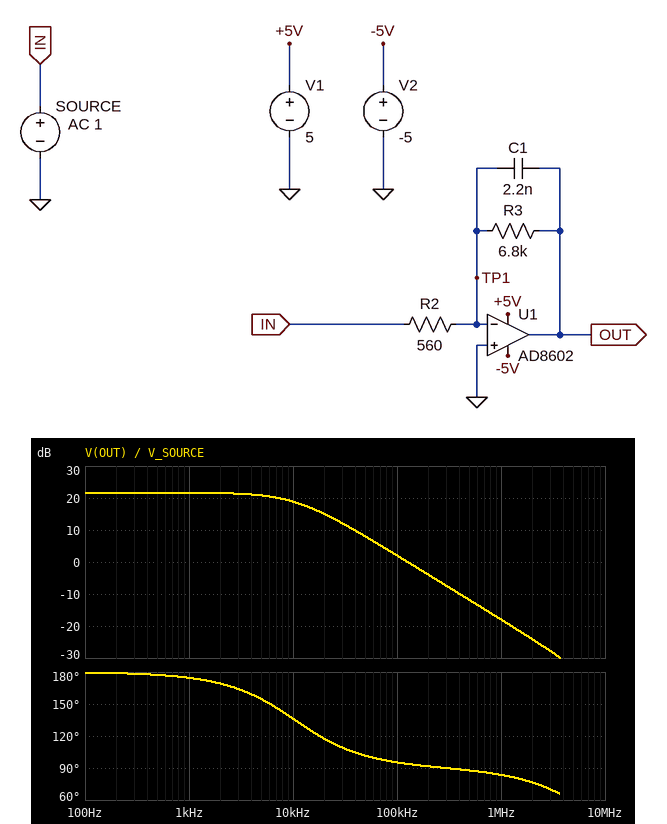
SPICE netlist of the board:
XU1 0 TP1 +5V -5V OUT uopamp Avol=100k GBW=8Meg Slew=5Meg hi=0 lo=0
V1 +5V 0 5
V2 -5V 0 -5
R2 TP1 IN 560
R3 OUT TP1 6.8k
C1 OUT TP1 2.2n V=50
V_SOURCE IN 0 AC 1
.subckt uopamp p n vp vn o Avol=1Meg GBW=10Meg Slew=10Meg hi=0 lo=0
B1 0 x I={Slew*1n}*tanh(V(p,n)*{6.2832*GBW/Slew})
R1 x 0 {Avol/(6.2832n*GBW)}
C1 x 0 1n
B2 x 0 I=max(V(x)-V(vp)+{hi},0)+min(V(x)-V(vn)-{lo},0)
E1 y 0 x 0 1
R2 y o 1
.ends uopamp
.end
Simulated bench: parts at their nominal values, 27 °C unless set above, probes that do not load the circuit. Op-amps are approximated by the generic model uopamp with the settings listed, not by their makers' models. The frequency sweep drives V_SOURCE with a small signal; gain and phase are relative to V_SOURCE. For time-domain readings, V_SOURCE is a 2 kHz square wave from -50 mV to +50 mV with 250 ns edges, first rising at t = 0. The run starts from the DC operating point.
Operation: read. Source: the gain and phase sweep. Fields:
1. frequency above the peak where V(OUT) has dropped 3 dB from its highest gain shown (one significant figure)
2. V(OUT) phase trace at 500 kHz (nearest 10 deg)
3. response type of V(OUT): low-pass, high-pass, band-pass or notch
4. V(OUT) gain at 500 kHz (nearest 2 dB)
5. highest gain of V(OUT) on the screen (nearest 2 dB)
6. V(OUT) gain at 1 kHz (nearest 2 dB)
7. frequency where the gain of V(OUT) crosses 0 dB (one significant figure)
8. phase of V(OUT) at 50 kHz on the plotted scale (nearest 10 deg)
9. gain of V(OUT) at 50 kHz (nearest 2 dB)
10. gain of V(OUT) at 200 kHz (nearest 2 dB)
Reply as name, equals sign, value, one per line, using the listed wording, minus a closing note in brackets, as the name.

frequency above the peak where V(OUT) has dropped 3 dB from its highest gain shown = 10 kHz
V(OUT) phase trace at 500 kHz = 90 deg
response type of V(OUT): low-pass, high-pass, band-pass or notch = low-pass
V(OUT) gain at 500 kHz = -12 dB
highest gain of V(OUT) on the screen = 22 dB
V(OUT) gain at 1 kHz = 22 dB
frequency where the gain of V(OUT) crosses 0 dB = 100 kHz
phase of V(OUT) at 50 kHz on the plotted scale = 100 deg
gain of V(OUT) at 50 kHz = 8 dB
gain of V(OUT) at 200 kHz = -4 dB
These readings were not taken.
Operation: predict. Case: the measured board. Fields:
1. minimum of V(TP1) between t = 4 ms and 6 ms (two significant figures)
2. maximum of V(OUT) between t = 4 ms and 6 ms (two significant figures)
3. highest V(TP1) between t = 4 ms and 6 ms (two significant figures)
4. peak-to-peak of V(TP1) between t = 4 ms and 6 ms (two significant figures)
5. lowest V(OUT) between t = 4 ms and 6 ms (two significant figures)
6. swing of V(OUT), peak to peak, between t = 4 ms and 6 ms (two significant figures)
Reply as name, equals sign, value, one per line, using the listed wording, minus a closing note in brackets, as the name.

minimum of V(TP1) between t = 4 ms and 6 ms = -1.6 mV
maximum of V(OUT) between t = 4 ms and 6 ms = 610 mV
highest V(TP1) between t = 4 ms and 6 ms = 1.6 mV
peak-to-peak of V(TP1) between t = 4 ms and 6 ms = 3.1 mV
lowest V(OUT) between t = 4 ms and 6 ms = -610 mV
swing of V(OUT), peak to peak, between t = 4 ms and 6 ms = 1.2 V
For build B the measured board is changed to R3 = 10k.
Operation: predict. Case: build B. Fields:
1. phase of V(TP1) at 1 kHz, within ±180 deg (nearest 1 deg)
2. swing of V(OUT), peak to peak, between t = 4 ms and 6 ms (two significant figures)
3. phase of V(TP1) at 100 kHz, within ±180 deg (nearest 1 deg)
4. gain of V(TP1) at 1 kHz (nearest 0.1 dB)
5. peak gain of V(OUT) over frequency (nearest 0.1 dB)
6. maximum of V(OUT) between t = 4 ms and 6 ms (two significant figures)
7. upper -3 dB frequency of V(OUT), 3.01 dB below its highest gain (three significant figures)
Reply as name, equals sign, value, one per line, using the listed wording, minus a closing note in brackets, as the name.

phase of V(TP1) at 1 kHz, within ±180 deg = 77 deg
swing of V(OUT), peak to peak, between t = 4 ms and 6 ms = 1.8 V
phase of V(TP1) at 100 kHz, within ±180 deg = 3 deg
gain of V(TP1) at 1 kHz = -53.1 dB
peak gain of V(OUT) over frequency = 25.0 dB
maximum of V(OUT) between t = 4 ms and 6 ms = 890 mV
upper -3 dB frequency of V(OUT), 3.01 dB below its highest gain = 7.12 kHz
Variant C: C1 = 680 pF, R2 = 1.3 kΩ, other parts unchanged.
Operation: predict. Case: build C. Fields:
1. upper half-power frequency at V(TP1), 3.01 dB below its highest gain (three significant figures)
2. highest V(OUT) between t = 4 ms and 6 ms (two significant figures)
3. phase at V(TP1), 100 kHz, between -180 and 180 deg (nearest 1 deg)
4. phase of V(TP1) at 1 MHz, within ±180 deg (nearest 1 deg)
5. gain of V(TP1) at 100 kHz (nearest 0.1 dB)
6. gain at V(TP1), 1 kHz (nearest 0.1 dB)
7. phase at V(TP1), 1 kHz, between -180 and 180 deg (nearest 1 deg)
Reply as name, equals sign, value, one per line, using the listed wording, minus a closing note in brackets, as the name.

upper half-power frequency at V(TP1), 3.01 dB below its highest gain = 8.25 MHz
highest V(OUT) between t = 4 ms and 6 ms = 260 mV
phase at V(TP1), 100 kHz, between -180 and 180 deg = 18 deg
phase of V(TP1) at 1 MHz, within ±180 deg = -5 deg
gain of V(TP1) at 100 kHz = -33.6 dB
gain at V(TP1), 1 kHz = -63.7 dB
phase at V(TP1), 1 kHz, between -180 and 180 deg = 84 deg
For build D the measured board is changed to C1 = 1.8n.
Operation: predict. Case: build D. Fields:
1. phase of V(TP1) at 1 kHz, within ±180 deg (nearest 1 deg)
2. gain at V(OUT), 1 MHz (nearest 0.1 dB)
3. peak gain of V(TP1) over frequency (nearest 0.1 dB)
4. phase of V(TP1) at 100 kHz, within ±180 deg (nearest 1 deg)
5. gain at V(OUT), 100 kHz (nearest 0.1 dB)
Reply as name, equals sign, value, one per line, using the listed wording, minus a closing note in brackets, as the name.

phase of V(TP1) at 1 kHz, within ±180 deg = 81 deg
gain at V(OUT), 1 MHz = -16.3 dB
peak gain of V(TP1) over frequency = -34.3 dB
phase of V(TP1) at 100 kHz, within ±180 deg = 7 deg
gain at V(OUT), 100 kHz = 3.7 dB
